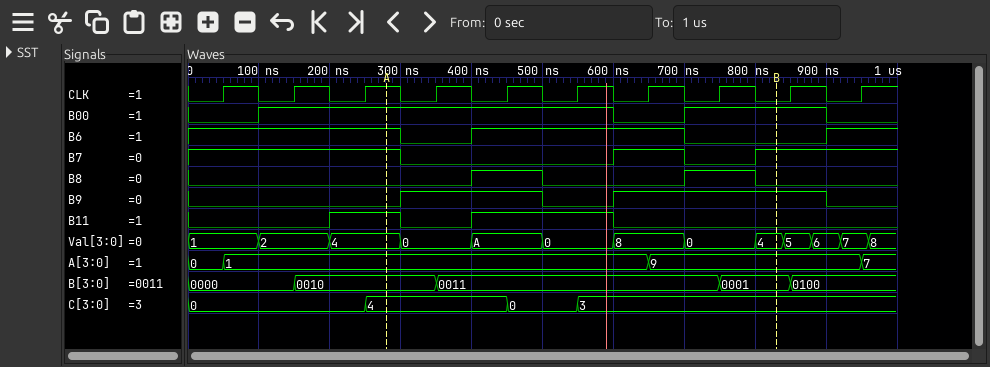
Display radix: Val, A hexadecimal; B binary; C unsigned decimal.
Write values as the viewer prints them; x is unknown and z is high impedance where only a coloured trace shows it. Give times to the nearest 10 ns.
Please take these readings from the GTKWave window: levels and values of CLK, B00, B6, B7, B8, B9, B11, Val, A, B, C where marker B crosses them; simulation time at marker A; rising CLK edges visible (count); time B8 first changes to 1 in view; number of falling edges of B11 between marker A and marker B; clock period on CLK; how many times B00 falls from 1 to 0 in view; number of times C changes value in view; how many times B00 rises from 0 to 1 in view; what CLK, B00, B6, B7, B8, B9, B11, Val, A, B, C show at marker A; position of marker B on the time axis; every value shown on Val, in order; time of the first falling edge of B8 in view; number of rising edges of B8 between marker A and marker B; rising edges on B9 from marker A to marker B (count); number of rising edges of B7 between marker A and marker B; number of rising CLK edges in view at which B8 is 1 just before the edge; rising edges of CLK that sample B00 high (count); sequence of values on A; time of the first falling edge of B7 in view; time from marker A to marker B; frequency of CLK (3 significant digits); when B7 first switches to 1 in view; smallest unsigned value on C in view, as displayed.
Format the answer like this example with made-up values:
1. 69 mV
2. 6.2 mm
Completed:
1. CLK=0, B00=1, B6=0, B7=1, B8=0, B9=1, B11=0, Val=4, A=9, B=0001, C=3
2. 280 ns
3. 10
4. 400 ns
5. 2
6. 100 ns
7. 2
8. 3
9. 2
10. CLK=1, B00=1, B6=1, B7=1, B8=0, B9=0, B11=1, Val=4, A=1, B=0010, C=4
11. 830 ns
12. 1, 2, 4, 0, A, 0, 8, 0, 4, 5, 6, 7, 8
13. 500 ns
14. 2
15. 2
16. 2
17. 2
18. 7
19. 0, 1, 9, 7
20. 300 ns
21. 550 ns
22. 10.0 MHz
23. 600 ns
24. 0
